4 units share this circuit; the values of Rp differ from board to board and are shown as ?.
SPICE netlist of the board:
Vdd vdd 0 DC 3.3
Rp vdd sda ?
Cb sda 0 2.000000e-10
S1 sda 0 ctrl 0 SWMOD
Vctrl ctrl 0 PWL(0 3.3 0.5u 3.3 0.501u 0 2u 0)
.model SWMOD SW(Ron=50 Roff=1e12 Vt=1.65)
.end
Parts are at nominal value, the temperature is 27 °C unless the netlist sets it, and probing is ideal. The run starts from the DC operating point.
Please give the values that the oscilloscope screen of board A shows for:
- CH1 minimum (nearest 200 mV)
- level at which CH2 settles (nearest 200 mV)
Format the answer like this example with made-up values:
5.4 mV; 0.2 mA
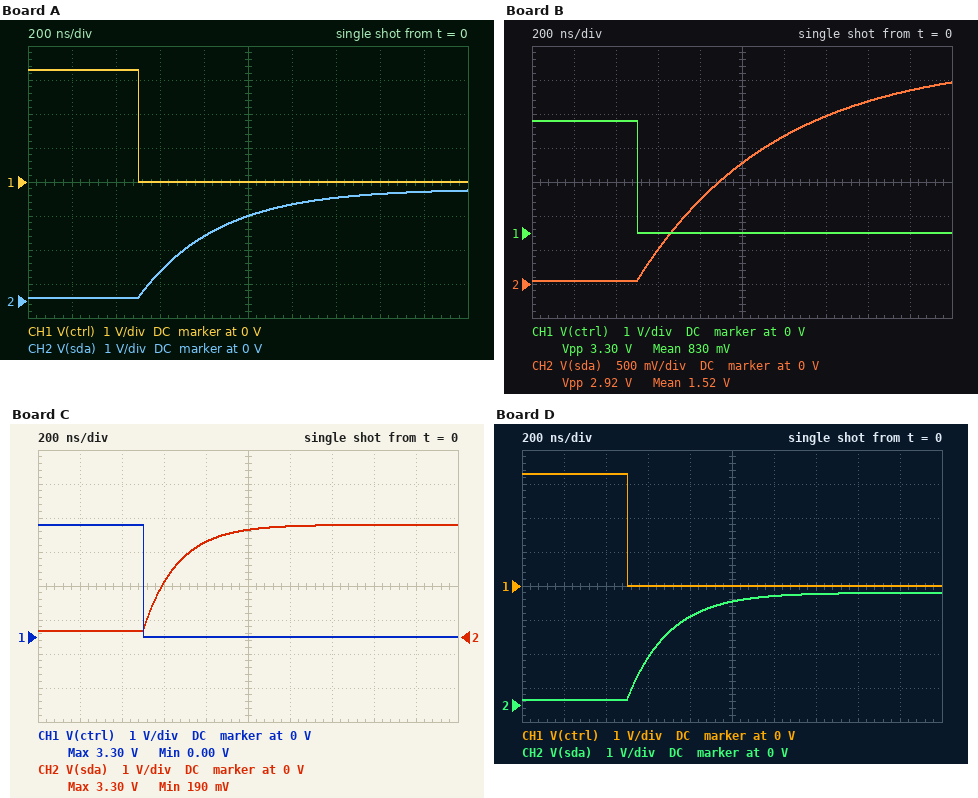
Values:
0 V; 3.2 V
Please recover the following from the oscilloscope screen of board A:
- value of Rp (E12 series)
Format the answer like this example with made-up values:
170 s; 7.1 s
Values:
1.8 kΩ
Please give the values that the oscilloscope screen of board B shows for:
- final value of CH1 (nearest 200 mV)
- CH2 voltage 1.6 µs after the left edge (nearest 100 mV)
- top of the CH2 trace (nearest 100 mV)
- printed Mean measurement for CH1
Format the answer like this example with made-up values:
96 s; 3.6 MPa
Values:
0 V; 2.7 V; 3.0 V; 830 mV
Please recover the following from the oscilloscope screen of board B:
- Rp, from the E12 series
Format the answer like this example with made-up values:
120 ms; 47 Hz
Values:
3.3 kΩ
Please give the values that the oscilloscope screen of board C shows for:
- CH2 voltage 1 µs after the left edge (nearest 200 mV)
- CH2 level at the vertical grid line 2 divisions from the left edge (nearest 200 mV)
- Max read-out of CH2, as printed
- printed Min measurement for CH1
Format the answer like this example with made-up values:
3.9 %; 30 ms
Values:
3.2 V; 200 mV; 3.30 V; 0.00 V
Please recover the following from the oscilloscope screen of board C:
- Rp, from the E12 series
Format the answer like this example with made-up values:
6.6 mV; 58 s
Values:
820 Ω
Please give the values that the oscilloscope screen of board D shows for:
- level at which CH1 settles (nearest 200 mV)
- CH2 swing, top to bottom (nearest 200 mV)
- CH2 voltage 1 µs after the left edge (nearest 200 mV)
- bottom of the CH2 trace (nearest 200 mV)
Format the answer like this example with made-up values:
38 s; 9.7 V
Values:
0 V; 3.2 V; 3.0 V; 200 mV
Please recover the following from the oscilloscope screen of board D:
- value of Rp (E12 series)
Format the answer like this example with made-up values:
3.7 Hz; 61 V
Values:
1 kΩ
